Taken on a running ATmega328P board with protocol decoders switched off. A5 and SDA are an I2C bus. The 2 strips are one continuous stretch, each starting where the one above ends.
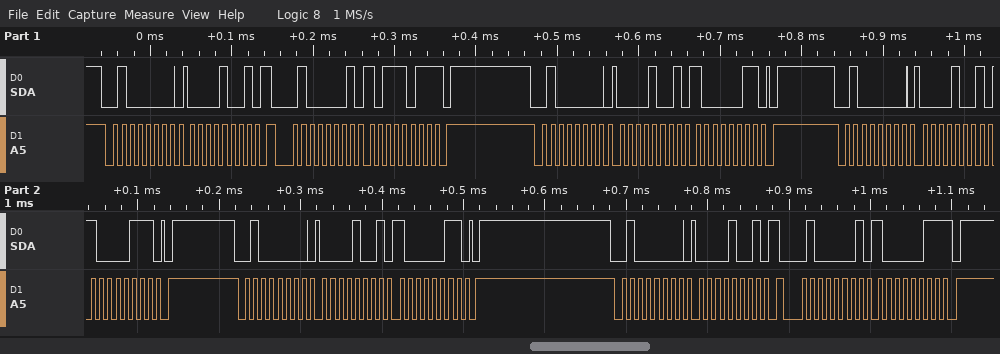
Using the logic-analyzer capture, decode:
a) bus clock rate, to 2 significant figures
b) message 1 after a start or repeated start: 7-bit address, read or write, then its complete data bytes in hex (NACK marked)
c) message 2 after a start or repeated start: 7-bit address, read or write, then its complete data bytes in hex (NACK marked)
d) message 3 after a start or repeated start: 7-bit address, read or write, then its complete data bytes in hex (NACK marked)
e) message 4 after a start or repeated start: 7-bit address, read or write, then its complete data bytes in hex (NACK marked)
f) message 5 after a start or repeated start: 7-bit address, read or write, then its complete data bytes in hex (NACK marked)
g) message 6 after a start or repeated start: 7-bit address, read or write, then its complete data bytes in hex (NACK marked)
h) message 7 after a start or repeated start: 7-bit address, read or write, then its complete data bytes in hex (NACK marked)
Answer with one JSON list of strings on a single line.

["100 kHz", "0x20 write: 09", "0x20 read: BB NACK", "0x20 write: 09 83", "0x20 write: 09 87", "0x20 write: 09 83", "0x20 write: 09", "0x20 read: 83 NACK"]
